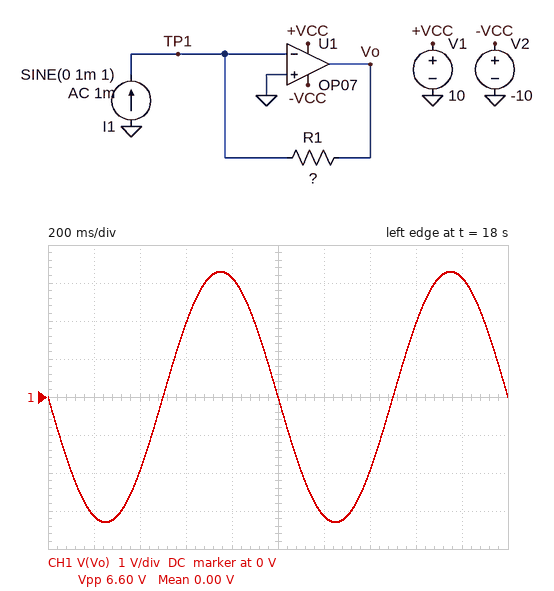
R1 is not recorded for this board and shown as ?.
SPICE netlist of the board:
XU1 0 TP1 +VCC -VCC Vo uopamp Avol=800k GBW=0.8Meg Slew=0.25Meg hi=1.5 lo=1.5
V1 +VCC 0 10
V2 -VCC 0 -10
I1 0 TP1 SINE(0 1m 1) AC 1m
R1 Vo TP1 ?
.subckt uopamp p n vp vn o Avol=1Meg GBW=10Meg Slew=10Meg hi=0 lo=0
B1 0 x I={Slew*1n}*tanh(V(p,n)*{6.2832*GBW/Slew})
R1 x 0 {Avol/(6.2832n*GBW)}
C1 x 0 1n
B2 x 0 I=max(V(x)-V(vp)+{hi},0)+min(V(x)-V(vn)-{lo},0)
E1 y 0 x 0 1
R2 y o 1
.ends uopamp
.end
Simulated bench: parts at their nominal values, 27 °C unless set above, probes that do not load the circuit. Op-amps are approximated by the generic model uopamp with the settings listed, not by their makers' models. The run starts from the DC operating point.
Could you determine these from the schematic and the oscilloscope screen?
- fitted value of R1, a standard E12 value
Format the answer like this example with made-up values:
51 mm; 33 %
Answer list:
3.3 kΩ
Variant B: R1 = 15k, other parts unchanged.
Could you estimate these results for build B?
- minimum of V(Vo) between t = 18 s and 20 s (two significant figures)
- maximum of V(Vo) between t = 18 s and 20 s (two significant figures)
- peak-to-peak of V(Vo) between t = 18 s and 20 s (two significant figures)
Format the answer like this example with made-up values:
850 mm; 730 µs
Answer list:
-8.5 V; 8.5 V; 17 V
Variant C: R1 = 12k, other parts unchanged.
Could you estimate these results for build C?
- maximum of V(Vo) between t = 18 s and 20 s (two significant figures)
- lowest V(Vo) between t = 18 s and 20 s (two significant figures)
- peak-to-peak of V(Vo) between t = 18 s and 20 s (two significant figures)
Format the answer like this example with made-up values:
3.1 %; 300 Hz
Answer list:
8.5 V; -8.5 V; 17 V
